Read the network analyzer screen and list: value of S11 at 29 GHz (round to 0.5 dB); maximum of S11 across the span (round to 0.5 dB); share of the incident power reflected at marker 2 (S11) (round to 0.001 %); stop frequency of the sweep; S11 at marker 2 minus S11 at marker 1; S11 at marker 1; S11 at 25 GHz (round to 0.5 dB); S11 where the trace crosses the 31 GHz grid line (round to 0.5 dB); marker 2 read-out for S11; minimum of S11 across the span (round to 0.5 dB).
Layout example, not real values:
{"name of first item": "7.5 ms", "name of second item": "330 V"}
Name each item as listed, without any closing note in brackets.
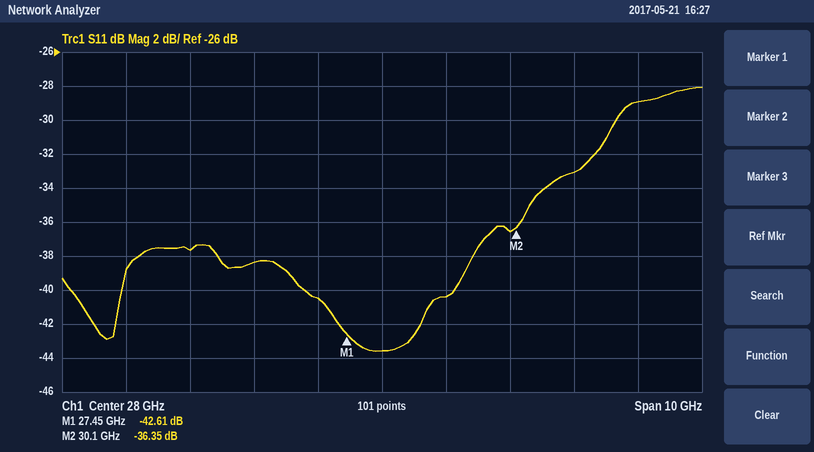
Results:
{"value of S11 at 29 GHz": "-40.5 dB", "maximum of S11 across the span": "-28.0 dB", "share of the incident power reflected at marker 2 (S11)": "0.023 %", "stop frequency of the sweep": "33 GHz", "S11 at marker 2 minus S11 at marker 1": "6.26 dB", "S11 at marker 1": "-42.61 dB", "S11 at 25 GHz": "-37.5 dB", "S11 where the trace crosses the 31 GHz grid line": "-33.0 dB", "marker 2 read-out for S11": "-36.35 dB", "minimum of S11 across the span": "-43.5 dB"}
